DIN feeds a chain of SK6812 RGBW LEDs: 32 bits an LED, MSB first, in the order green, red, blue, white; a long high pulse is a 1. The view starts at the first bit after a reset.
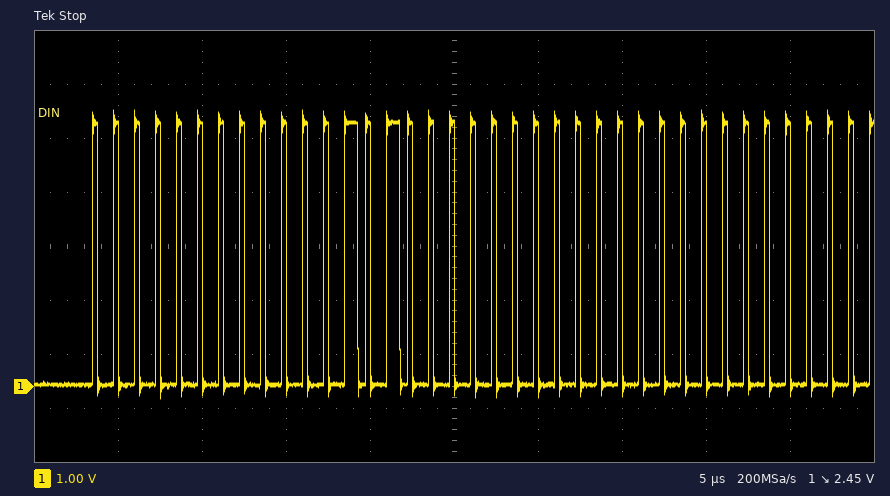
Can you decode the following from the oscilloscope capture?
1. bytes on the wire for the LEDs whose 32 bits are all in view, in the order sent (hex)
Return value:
00 0A 00 00
